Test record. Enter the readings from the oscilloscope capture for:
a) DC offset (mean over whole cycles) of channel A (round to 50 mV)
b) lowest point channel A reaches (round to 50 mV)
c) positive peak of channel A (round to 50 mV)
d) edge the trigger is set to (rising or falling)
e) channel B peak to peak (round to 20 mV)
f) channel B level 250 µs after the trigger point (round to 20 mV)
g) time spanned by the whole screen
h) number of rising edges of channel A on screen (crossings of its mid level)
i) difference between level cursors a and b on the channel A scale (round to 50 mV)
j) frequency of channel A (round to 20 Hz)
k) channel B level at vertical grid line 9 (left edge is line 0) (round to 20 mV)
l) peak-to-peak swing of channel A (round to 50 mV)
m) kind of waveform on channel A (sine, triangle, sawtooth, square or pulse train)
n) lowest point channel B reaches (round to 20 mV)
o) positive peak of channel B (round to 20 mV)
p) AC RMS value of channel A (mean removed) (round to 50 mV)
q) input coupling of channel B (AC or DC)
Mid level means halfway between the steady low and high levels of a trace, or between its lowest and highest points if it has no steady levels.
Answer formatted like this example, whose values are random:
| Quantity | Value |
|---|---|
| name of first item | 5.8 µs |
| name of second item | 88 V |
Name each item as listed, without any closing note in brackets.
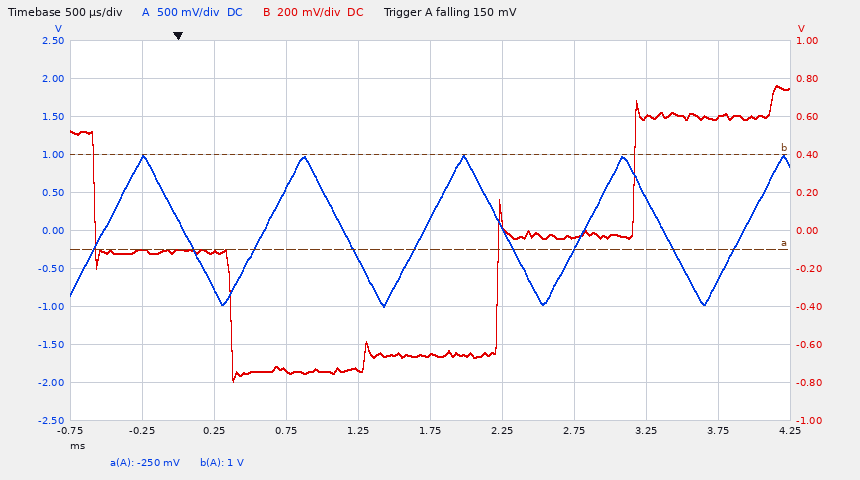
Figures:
| Quantity | Value |
|---|---|
| DC offset (mean over whole cycles) of channel A | 0 mV |
| lowest point channel A reaches | -1.00 V |
| positive peak of channel A | 1.00 V |
| edge the trigger is set to | falling |
| channel B peak to peak | 1.56 V |
| channel B level 250 µs after the trigger point | -120 mV |
| time spanned by the whole screen | 5 ms |
| number of rising edges of channel A on screen | 5 |
| difference between level cursors a and b on the channel A scale | 1.25 V |
| frequency of channel A | 900 Hz |
| channel B level at vertical grid line 9 (left edge is line 0) | 600 mV |
| peak-to-peak swing of channel A | 2.00 V |
| kind of waveform on channel A | triangle |
| lowest point channel B reaches | -800 mV |
| positive peak of channel B | 760 mV |
| AC RMS value of channel A (mean removed) | 600 mV |
| input coupling of channel B | DC |
